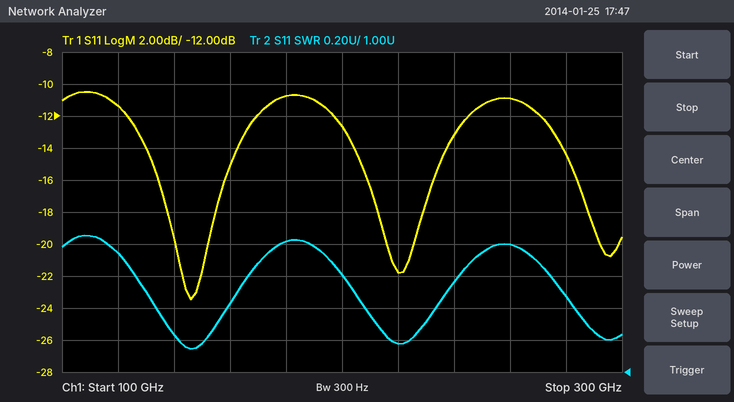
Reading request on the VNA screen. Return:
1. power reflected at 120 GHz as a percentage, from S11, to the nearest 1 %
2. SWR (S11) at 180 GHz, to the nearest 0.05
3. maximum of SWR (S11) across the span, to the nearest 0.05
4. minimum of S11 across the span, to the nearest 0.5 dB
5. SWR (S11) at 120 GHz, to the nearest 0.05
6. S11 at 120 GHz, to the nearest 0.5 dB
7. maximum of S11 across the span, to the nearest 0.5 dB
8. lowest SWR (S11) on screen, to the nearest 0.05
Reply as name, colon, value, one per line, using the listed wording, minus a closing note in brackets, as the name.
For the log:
power reflected at 120 GHz as a percentage, from S11, to the nearest 1 %: 7 %
SWR (S11) at 180 GHz, to the nearest 0.05: 1.80
maximum of SWR (S11) across the span, to the nearest 0.05: 1.85
minimum of S11 across the span, to the nearest 0.5 dB: -23.5 dB
SWR (S11) at 120 GHz, to the nearest 0.05: 1.75
S11 at 120 GHz, to the nearest 0.5 dB: -11.5 dB
maximum of S11 across the span, to the nearest 0.5 dB: -10.5 dB
lowest SWR (S11) on screen, to the nearest 0.05: 1.15
